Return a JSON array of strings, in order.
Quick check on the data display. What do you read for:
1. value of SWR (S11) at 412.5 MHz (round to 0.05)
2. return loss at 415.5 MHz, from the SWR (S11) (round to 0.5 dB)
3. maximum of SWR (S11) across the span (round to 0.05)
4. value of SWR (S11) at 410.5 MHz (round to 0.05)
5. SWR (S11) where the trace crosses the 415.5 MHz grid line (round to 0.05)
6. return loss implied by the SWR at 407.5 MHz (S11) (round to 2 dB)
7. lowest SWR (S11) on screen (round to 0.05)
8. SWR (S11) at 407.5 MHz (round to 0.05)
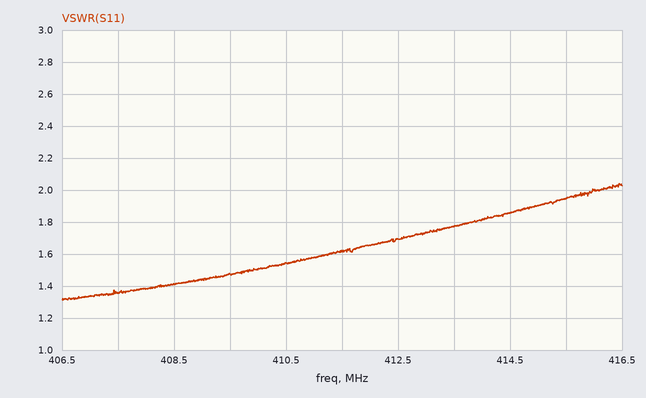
["1.70", "10.0 dB", "2.05", "1.55", "1.95", "16 dB", "1.30", "1.35"]
